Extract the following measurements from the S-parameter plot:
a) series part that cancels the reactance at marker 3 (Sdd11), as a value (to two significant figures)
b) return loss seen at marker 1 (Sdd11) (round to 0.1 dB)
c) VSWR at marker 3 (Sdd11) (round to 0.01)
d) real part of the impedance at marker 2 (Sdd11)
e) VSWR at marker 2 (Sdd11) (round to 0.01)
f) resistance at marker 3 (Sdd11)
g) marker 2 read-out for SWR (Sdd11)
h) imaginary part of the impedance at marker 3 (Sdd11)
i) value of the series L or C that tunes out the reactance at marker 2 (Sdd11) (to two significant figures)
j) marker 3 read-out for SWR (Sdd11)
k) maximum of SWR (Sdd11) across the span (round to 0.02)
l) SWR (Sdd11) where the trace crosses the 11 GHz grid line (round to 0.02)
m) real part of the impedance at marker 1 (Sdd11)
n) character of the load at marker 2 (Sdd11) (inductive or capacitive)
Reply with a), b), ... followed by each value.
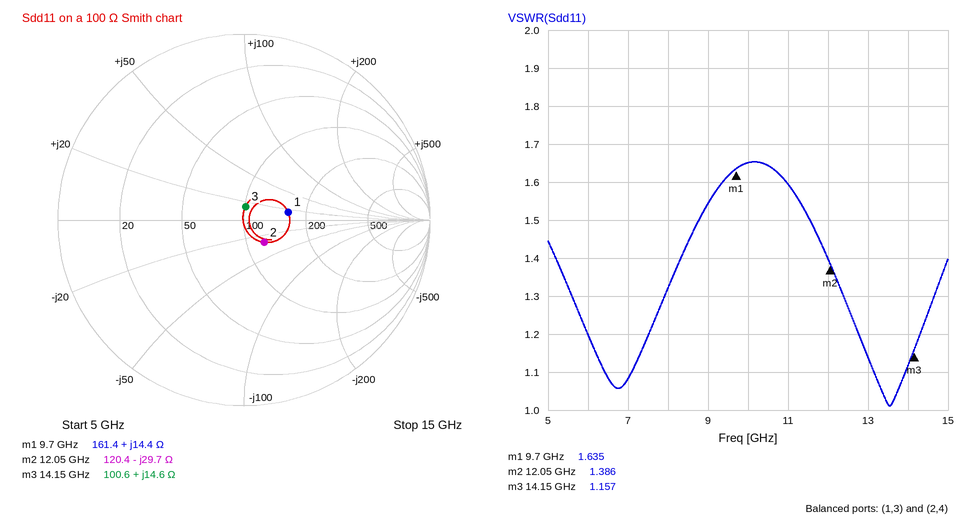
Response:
a) 770 fF
b) 12.4 dB
c) 1.16
d) 120.4 Ω
e) 1.39
f) 100.6 Ω
g) 1.386
h) +14.6 Ω
i) 390 pH
j) 1.157
k) 1.66
l) 1.60
m) 161.4 Ω
n) capacitive
